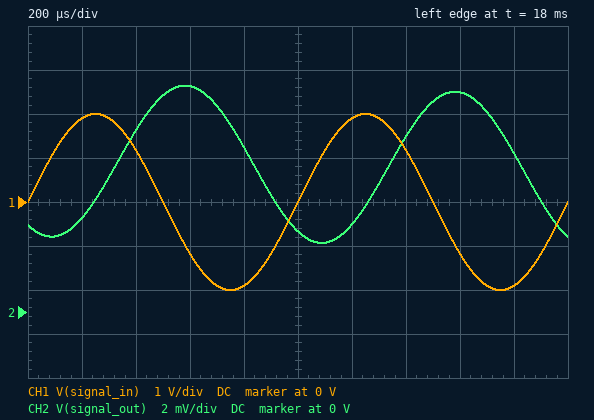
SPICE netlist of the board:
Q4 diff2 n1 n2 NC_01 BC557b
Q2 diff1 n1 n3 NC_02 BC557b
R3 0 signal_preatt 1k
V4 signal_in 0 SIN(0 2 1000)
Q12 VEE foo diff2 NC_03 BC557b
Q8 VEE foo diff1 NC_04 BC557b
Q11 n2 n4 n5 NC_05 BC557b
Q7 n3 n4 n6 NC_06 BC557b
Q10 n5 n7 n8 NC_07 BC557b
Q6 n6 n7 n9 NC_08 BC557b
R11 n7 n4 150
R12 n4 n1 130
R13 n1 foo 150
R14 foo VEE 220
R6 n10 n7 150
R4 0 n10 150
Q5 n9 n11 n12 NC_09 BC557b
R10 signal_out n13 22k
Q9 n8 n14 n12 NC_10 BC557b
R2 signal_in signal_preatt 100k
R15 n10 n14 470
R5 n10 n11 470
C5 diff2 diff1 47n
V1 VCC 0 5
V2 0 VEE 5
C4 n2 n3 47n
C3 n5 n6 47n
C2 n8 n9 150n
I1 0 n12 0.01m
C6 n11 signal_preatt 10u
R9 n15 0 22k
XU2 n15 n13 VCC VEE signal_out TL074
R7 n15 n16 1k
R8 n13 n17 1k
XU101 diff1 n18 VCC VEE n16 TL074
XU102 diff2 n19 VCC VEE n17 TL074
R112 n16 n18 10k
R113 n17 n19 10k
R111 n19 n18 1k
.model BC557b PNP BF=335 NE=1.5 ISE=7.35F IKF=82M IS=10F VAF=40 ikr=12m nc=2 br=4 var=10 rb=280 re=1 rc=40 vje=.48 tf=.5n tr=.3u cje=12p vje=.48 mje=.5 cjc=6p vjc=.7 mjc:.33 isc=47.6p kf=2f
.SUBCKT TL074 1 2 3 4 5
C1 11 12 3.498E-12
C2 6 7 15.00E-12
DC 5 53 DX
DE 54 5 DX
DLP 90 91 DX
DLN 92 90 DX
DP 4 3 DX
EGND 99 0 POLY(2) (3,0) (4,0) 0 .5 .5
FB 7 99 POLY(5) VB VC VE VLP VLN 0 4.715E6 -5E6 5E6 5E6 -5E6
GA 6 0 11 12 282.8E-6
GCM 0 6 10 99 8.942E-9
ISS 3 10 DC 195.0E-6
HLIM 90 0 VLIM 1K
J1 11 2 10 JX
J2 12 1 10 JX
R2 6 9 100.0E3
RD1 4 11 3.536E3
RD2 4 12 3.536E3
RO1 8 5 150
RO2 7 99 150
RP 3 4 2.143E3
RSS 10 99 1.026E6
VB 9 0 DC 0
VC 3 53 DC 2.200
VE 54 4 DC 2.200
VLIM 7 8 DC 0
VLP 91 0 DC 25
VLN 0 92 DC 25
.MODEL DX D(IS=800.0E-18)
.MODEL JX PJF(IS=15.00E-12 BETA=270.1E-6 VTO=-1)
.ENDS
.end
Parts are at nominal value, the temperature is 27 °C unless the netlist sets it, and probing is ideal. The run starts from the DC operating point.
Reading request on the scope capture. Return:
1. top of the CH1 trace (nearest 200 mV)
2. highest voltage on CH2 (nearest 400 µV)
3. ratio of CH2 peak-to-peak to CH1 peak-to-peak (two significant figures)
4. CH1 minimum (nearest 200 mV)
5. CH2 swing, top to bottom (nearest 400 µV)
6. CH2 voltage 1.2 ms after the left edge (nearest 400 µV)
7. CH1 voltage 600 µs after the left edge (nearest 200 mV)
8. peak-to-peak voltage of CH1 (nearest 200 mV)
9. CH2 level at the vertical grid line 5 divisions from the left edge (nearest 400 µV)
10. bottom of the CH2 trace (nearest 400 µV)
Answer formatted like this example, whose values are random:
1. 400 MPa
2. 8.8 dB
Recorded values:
1. 2.0 V
2. 10.4 mV
3. 0.0018
4. -2.0 V
5. 7.2 mV
6. 4.0 mV
7. -1.2 V
8. 4.0 V
9. 3.6 mV
10. 3.2 mV
